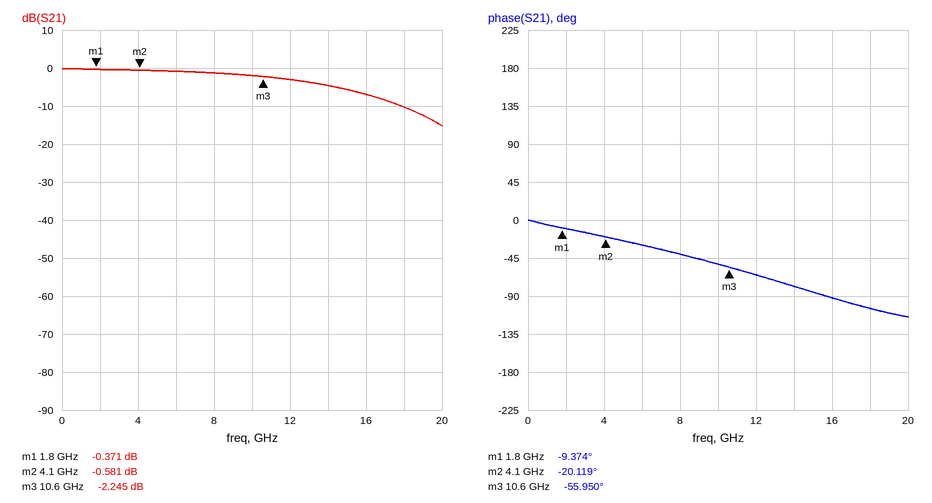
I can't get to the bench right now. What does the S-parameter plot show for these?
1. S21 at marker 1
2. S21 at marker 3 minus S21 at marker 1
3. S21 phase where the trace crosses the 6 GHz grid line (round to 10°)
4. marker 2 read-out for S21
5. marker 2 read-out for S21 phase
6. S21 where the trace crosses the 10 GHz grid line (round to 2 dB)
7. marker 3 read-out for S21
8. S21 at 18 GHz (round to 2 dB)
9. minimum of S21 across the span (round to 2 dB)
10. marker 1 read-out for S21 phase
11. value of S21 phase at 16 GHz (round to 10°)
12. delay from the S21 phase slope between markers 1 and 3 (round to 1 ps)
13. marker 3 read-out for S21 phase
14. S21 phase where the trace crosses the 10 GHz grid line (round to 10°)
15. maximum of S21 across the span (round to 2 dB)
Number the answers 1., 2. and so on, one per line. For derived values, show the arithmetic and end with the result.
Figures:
1. -0.371 dB
2. -2.245 − (-0.371) = -1.874 dB
3. -30°
4. -0.581 dB
5. -20.119°
6. -2 dB
7. -2.245 dB
8. -10 dB
9. -16 dB
10. -9.374°
11. -90°
12. −(-55.95° − (-9.374°))/(360° × 8.8 GHz) ≈ 15 ps
13. -55.950°
14. -50°
15. 0 dB
